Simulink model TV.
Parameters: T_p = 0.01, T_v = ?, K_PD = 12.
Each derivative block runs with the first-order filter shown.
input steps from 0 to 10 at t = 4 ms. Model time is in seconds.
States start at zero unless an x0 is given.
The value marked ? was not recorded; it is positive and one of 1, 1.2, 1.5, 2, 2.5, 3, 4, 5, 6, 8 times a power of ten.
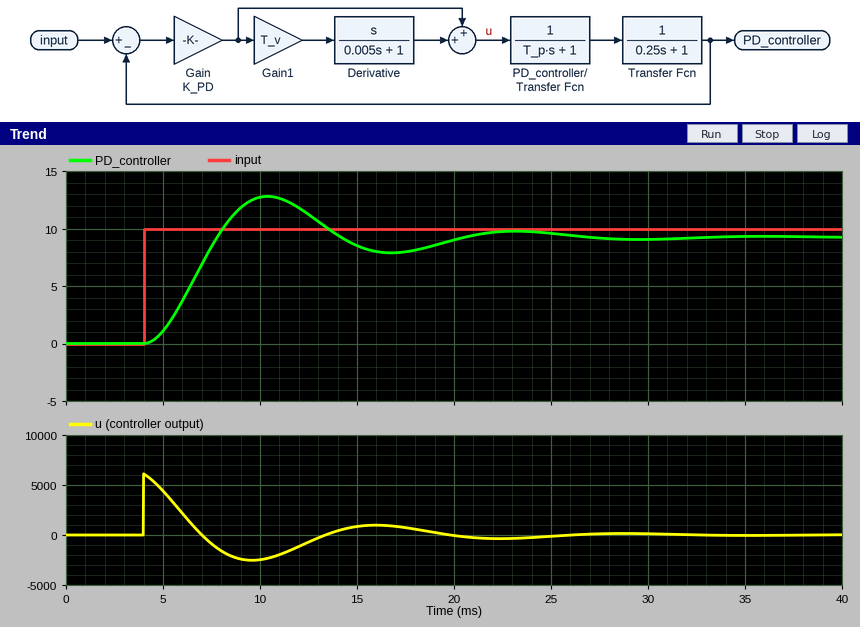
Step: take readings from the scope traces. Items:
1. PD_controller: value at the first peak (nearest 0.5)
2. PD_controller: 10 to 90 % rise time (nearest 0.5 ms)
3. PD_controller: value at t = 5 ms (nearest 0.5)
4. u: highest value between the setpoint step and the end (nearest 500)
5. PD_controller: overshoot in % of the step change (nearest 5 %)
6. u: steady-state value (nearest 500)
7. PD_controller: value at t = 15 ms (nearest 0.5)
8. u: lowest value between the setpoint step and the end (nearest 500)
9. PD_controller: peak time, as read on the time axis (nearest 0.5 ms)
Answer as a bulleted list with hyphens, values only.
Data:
- 13.0
- 2.5 ms
- 1.0
- 6000
- 40 %
- 0
- 8.5
- -2500
- 10.5 ms
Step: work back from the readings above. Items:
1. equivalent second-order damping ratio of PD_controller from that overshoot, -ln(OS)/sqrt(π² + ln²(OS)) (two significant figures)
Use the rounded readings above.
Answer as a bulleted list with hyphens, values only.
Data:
- 0.28
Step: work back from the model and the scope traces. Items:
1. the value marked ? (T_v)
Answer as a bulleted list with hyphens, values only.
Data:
- 0.25
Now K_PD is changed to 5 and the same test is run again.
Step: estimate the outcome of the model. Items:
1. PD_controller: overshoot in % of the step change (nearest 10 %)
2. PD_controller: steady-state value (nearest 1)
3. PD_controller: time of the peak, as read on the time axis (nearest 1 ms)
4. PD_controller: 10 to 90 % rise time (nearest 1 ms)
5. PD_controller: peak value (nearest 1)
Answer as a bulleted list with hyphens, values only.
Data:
- 20 %
- 8
- 14 ms
- 4 ms
- 10
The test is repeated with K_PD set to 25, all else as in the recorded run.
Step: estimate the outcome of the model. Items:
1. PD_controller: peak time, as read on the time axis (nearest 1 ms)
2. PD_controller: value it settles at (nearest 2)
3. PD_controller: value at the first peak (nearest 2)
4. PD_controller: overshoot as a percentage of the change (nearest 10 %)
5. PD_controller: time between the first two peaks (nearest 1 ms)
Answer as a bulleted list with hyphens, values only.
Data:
- 8 ms
- 10
- 14
- 50 %
- 9 ms
